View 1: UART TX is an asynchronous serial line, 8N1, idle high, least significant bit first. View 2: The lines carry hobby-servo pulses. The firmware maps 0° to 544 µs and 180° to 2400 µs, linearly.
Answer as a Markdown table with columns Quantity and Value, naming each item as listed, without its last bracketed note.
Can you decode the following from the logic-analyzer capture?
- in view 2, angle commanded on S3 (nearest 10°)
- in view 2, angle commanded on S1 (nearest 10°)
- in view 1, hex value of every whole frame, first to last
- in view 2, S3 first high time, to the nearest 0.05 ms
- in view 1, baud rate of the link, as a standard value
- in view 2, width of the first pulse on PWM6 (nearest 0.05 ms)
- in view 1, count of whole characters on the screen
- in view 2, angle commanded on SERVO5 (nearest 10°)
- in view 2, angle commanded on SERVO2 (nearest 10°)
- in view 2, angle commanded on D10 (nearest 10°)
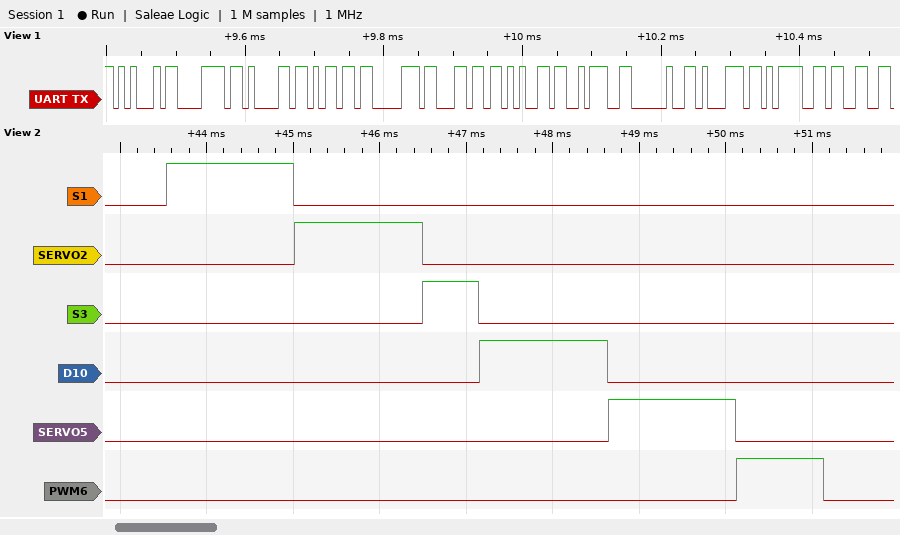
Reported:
| Quantity | Value |
|---|---|
| in view 2, angle commanded on S3 | 10° |
| in view 2, angle commanded on S1 | 90° |
| in view 1, hex value of every whole frame, first to last | 45 78 61 6D 70 6C 65 3A 20 71 3D 33 |
| in view 2, S3 first high time, to the nearest 0.05 ms | 0.65 ms |
| in view 1, baud rate of the link, as a standard value | 115200 baud |
| in view 2, width of the first pulse on PWM6 | 1.00 ms |
| in view 1, count of whole characters on the screen | 12 |
| in view 2, angle commanded on SERVO5 | 90° |
| in view 2, angle commanded on SERVO2 | 90° |
| in view 2, angle commanded on D10 | 90° |
